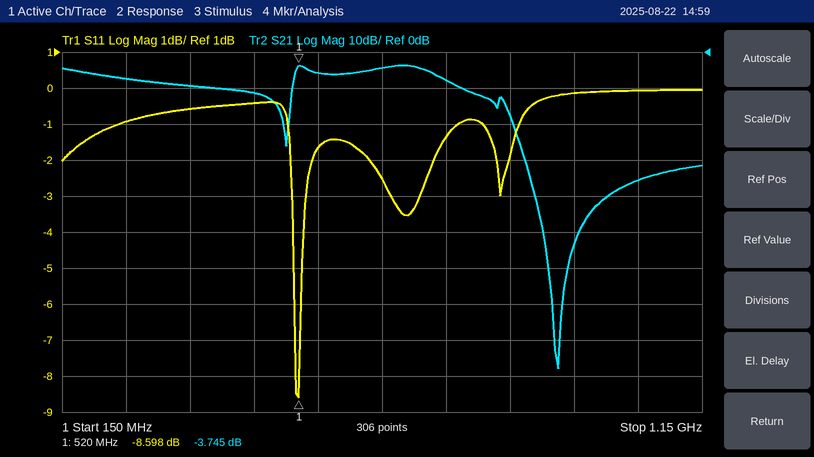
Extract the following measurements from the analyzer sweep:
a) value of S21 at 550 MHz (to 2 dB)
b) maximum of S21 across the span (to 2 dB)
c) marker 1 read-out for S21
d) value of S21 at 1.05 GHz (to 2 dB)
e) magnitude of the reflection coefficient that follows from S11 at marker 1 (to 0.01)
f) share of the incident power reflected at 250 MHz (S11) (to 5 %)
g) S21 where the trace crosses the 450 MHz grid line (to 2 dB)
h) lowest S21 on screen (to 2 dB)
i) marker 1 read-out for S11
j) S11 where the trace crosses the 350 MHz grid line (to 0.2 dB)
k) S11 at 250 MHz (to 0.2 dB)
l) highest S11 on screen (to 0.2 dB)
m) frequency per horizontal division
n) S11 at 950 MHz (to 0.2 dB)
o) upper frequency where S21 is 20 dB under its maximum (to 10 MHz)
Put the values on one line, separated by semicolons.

-6 dB; -4 dB; -3.745 dB; -36 dB; 0.37; 80 %; -12 dB; -88 dB; -8.598 dB; -0.6 dB; -1.0 dB; 0.0 dB; 100 MHz; -0.2 dB; 860 MHz
